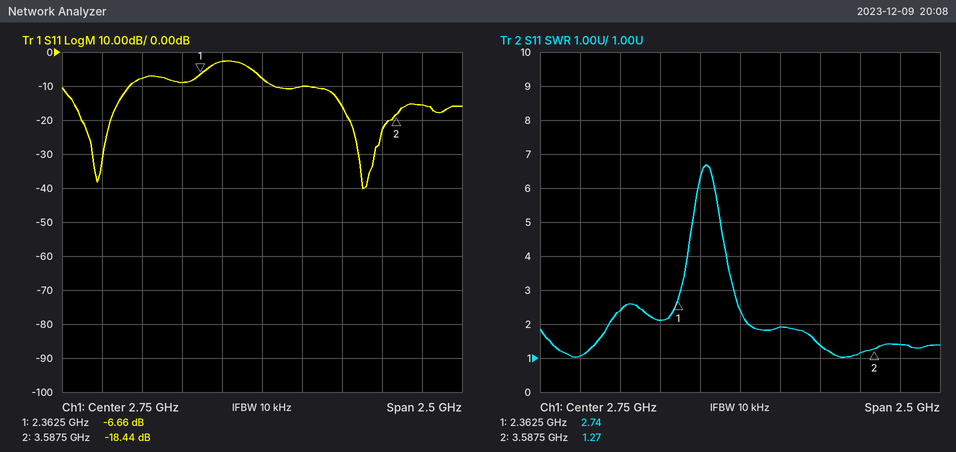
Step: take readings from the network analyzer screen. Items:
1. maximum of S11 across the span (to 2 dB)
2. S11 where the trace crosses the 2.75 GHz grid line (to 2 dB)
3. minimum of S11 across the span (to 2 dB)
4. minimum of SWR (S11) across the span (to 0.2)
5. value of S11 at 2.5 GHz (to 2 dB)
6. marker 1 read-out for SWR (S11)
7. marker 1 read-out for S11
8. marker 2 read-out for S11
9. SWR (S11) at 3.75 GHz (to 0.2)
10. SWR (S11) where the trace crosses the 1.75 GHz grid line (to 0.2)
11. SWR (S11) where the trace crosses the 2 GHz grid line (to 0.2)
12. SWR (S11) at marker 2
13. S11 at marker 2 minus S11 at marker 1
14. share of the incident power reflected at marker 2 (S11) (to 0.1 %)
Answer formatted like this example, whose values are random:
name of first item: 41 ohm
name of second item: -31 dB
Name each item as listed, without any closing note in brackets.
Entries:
maximum of S11 across the span: -2 dB
S11 where the trace crosses the 2.75 GHz grid line: -8 dB
minimum of S11 across the span: -40 dB
minimum of SWR (S11) across the span: 1.0
value of S11 at 2.5 GHz: -2 dB
marker 1 read-out for SWR: 2.74
marker 1 read-out for S11: -6.66 dB
marker 2 read-out for S11: -18.44 dB
SWR (S11) at 3.75 GHz: 1.4
SWR (S11) where the trace crosses the 1.75 GHz grid line: 1.0
SWR (S11) where the trace crosses the 2 GHz grid line: 2.4
SWR (S11) at marker 2: 1.27
S11 at marker 2 minus S11 at marker 1: -11.78 dB
share of the incident power reflected at marker 2 (S11): 1.4 %
